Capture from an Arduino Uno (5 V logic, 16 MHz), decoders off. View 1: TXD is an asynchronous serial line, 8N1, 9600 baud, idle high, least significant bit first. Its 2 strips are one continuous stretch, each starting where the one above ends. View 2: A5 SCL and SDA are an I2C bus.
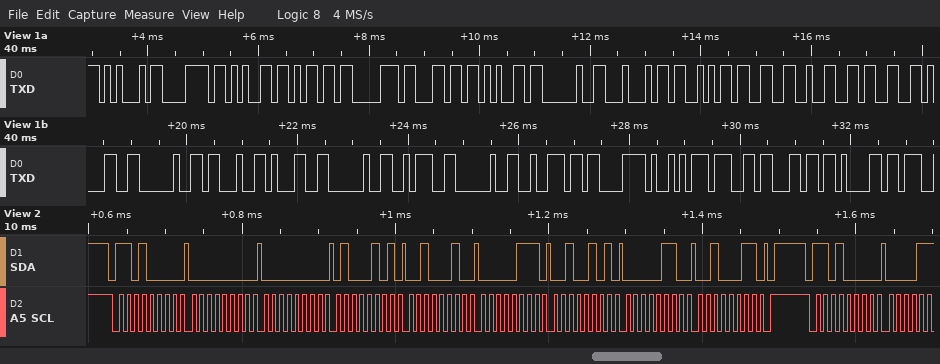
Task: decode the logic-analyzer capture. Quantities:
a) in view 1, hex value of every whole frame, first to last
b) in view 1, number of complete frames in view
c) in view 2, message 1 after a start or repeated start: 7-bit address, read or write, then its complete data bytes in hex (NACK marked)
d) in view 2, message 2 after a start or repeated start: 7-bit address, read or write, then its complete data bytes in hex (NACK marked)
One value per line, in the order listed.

45 78 65 6D 70 6C 65 20 44 53 33 32 33 31 20 23 31 20 3A 20 72 C3 A9 67 6C 61
26
0x68 write: 00 00 45 22 07 25 06 23
0x68 write
